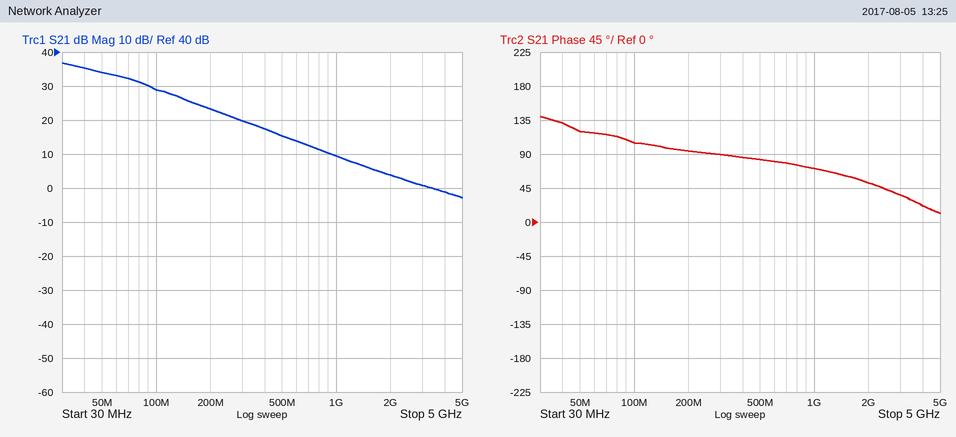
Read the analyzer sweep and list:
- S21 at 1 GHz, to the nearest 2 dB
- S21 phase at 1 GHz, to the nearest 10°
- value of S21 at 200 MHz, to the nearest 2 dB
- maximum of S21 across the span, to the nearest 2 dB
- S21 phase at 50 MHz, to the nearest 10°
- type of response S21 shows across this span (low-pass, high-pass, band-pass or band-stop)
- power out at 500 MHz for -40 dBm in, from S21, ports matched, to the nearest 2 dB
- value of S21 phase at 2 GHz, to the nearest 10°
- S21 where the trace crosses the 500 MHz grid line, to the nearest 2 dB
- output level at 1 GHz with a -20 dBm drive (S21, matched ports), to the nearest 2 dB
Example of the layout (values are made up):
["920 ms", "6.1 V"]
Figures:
["10 dB", "70°", "24 dB", "36 dB", "120°", "low-pass", "-24 dBm", "50°", "16 dB", "-10 dBm"]
